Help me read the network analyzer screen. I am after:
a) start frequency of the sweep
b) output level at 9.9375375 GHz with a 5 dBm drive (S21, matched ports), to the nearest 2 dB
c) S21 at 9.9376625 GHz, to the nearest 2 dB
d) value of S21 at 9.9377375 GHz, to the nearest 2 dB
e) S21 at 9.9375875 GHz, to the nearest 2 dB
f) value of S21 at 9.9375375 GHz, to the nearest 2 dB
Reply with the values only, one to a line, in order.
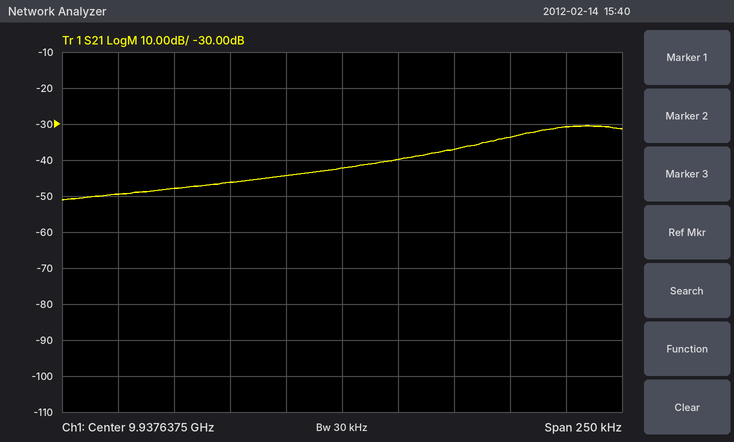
9.9375125 GHz
-44 dBm
-40 dB
-30 dB
-46 dB
-50 dB
